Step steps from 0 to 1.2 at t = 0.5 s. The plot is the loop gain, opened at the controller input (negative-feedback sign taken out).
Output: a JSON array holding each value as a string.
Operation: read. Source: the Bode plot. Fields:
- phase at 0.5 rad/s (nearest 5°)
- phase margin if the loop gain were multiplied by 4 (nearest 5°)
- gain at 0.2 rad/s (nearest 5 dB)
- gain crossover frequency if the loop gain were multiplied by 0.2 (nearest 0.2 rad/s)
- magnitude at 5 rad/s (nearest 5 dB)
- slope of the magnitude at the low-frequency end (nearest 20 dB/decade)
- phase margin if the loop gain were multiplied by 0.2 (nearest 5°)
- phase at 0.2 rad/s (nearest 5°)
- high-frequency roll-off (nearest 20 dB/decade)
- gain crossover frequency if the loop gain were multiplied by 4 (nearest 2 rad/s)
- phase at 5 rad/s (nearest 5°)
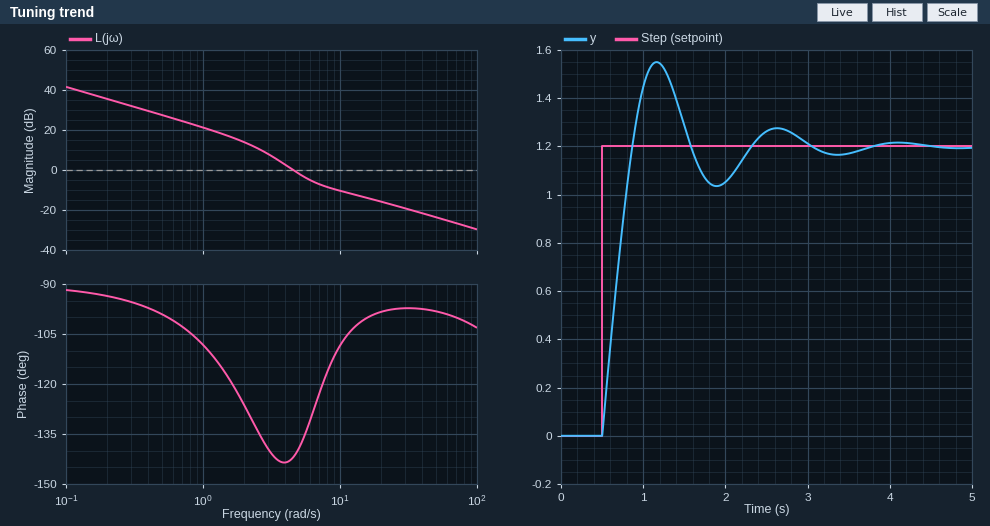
["-100°", "75°", "35 dB", "2.0 rad/s", "0 dB", "-20 dB/decade", "55°", "-95°", "-20 dB/decade", "12 rad/s", "-140°"]
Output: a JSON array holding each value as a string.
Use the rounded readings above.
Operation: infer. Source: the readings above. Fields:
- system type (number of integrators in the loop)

["1"]
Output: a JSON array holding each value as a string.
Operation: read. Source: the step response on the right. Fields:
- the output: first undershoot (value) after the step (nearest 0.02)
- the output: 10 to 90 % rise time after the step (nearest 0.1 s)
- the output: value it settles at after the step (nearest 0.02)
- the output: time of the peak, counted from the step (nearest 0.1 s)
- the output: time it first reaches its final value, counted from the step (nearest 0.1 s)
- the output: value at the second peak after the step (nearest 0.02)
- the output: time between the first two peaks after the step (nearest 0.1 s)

["1.04", "0.3 s", "1.20", "0.7 s", "0.4 s", "1.28", "1.5 s"]
